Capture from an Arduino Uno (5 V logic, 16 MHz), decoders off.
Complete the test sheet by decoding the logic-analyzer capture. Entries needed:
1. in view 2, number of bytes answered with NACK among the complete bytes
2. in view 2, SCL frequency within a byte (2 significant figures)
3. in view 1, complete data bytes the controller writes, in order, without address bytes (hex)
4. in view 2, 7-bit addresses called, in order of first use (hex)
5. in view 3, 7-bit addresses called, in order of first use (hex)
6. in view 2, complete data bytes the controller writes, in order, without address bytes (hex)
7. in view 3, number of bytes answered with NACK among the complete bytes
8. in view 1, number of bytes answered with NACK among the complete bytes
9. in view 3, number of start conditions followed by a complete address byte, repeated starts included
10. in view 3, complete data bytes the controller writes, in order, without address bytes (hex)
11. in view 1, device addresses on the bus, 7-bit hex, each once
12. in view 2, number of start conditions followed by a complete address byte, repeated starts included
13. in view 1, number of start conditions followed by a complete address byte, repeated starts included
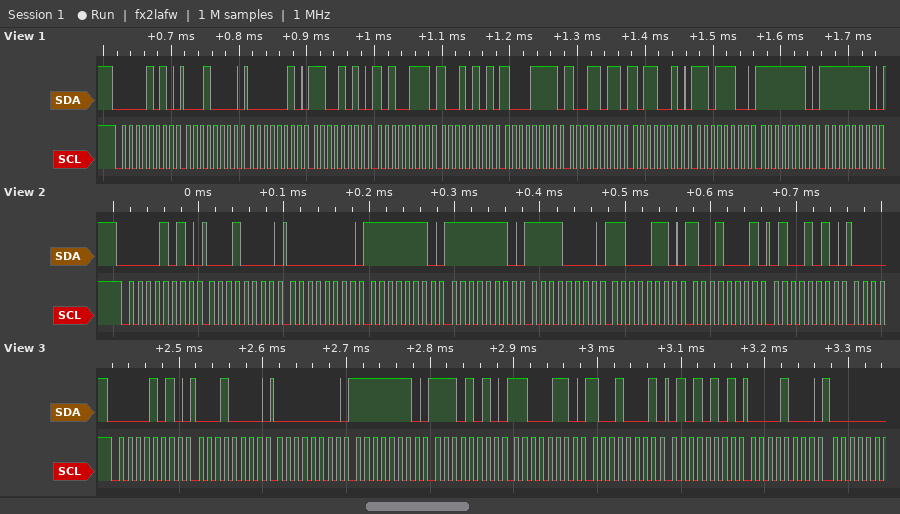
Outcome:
0
100 kHz
10 02 CA A7 95 8F 9B B2 DC FE FE
0x05
0x05
10 00 FE FE F0 C6 91 4A
0
0
1
10 00 FE EA C6 91 55 08
0x05
1
1
